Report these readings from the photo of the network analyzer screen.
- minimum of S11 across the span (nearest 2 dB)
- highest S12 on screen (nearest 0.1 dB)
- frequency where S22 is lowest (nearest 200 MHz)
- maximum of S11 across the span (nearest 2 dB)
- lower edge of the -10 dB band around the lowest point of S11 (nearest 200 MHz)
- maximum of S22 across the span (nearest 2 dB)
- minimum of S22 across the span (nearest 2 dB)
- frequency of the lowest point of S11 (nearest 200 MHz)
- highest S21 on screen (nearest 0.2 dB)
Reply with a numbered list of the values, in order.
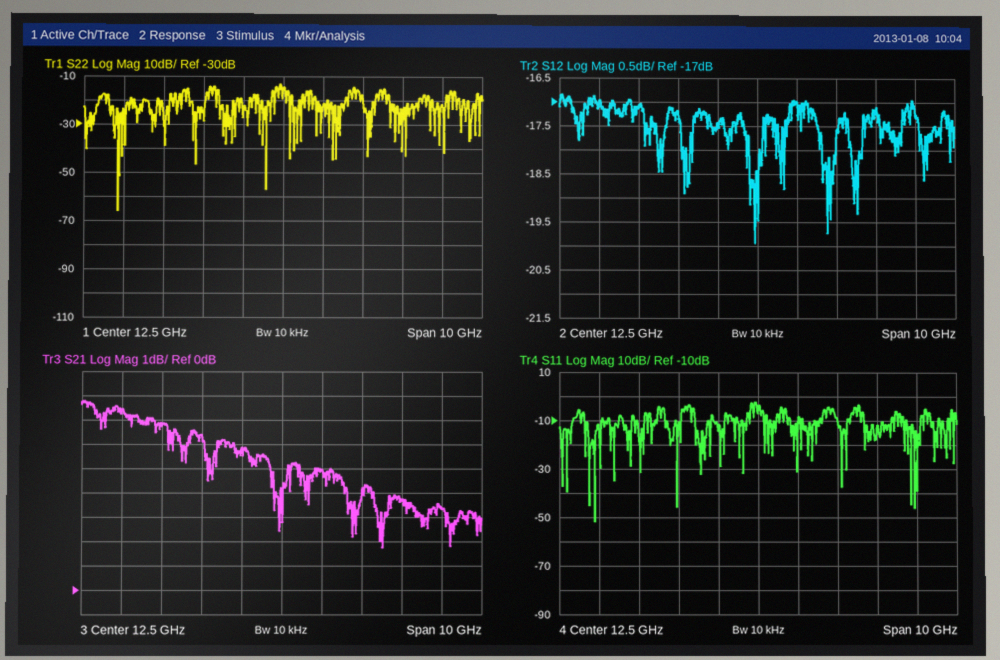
1. -52 dB
2. -16.8 dB
3. 8.4 GHz
4. -2 dB
5. 8.2 GHz
6. -14 dB
7. -66 dB
8. 8.4 GHz
9. 7.8 dB
